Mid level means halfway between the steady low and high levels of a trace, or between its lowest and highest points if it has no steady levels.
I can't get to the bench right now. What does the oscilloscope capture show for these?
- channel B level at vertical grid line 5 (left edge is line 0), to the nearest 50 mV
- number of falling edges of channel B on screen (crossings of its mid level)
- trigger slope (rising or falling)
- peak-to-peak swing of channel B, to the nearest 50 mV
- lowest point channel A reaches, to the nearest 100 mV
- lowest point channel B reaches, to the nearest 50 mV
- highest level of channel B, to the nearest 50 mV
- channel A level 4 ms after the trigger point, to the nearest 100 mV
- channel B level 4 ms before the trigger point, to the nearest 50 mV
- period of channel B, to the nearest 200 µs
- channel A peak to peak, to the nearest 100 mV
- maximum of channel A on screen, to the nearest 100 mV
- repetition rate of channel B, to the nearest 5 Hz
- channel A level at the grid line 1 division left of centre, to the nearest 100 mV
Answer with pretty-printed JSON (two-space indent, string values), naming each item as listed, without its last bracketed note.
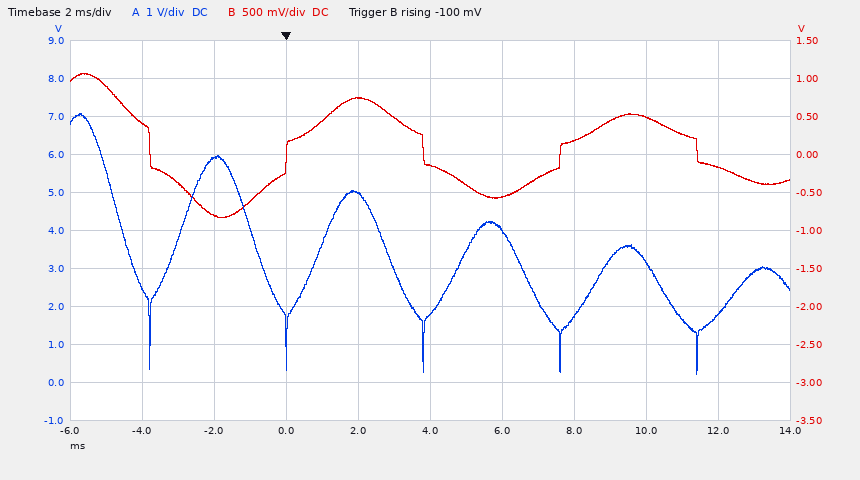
{
  "channel B level at vertical grid line 5 (left edge is line 0), to the nearest 50 mV": "-150 mV",
  "number of falling edges of channel B on screen": "3",
  "trigger slope": "rising",
  "peak-to-peak swing of channel B, to the nearest 50 mV": "1.90 V",
  "lowest point channel A reaches, to the nearest 100 mV": "200 mV",
  "lowest point channel B reaches, to the nearest 50 mV": "-850 mV",
  "highest level of channel B, to the nearest 50 mV": "1.05 V",
  "channel A level 4 ms after the trigger point, to the nearest 100 mV": "1.8 V",
  "channel B level 4 ms before the trigger point, to the nearest 50 mV": "400 mV",
  "period of channel B, to the nearest 200 µs": "7.6 ms",
  "channel A peak to peak, to the nearest 100 mV": "6.9 V",
  "maximum of channel A on screen, to the nearest 100 mV": "7.1 V",
  "repetition rate of channel B, to the nearest 5 Hz": "130 Hz",
  "channel A level at the grid line 1 division left of centre, to the nearest 100 mV": "5.0 V"
}
